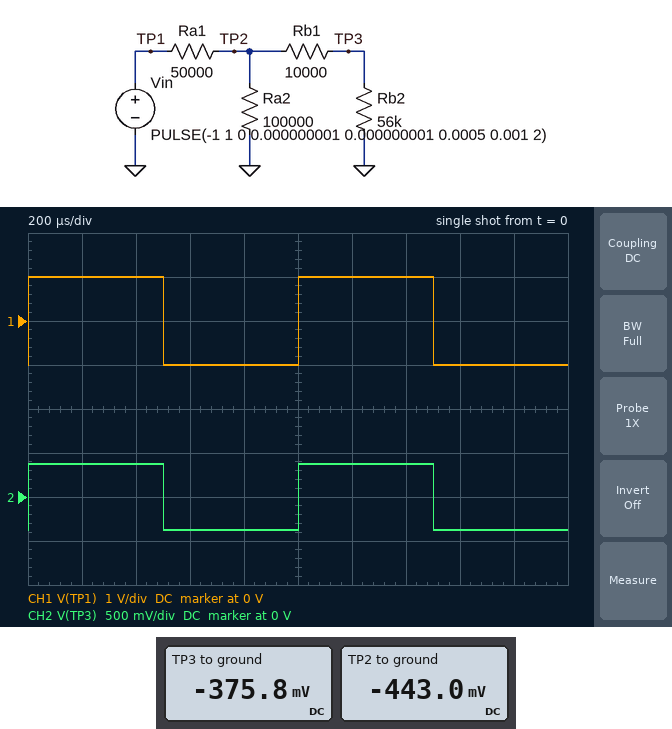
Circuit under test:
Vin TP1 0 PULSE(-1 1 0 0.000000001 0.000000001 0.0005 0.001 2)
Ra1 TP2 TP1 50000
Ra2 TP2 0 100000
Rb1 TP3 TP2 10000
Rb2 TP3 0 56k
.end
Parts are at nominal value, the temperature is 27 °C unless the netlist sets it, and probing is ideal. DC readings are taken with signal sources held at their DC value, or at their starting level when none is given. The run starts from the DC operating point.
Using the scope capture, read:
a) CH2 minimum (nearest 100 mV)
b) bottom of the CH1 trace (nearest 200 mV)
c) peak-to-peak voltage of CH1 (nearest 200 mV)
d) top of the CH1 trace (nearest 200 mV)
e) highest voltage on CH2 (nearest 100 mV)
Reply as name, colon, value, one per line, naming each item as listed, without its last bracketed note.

CH2 minimum: -400 mV
bottom of the CH1 trace: -1.0 V
peak-to-peak voltage of CH1: 2.0 V
top of the CH1 trace: 1.0 V
highest voltage on CH2: 400 mV
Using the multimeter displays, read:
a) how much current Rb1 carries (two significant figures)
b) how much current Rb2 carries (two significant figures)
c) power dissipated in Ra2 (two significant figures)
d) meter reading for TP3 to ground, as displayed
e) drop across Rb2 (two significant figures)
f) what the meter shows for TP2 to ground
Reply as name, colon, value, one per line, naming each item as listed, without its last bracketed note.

how much current Rb1 carries: 6.7 µA
how much current Rb2 carries: 6.7 µA
power dissipated in Ra2: 2.0 µW
meter reading for TP3 to ground, as displayed: -375.8 mV
drop across Rb2: 380 mV
what the meter shows for TP2 to ground: -443.0 mV
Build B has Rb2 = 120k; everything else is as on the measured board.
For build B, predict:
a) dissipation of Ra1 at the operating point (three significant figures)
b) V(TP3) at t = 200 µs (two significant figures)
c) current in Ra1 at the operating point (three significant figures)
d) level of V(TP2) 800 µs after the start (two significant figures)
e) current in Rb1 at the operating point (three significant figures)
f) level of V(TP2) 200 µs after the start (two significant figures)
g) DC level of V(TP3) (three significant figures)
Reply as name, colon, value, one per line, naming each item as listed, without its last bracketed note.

dissipation of Ra1 at the operating point: 4.41 µW
V(TP3) at t = 200 µs: 490 mV
current in Ra1 at the operating point: 9.39 µA
level of V(TP2) 800 µs after the start: -530 mV
current in Rb1 at the operating point: 4.08 µA
level of V(TP2) 200 µs after the start: 530 mV
DC level of V(TP3): -490 mV
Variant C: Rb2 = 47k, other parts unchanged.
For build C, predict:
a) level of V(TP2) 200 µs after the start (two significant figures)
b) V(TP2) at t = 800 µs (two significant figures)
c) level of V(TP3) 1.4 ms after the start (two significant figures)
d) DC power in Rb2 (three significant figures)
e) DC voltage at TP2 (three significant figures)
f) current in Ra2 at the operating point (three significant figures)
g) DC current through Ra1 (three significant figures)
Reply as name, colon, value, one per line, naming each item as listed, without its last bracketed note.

level of V(TP2) 200 µs after the start: 420 mV
V(TP2) at t = 800 µs: -420 mV
level of V(TP3) 1.4 ms after the start: 350 mV
DC power in Rb2: 2.56 µW
DC voltage at TP2: -421 mV
current in Ra2 at the operating point: 4.21 µA
DC current through Ra1: 11.6 µA
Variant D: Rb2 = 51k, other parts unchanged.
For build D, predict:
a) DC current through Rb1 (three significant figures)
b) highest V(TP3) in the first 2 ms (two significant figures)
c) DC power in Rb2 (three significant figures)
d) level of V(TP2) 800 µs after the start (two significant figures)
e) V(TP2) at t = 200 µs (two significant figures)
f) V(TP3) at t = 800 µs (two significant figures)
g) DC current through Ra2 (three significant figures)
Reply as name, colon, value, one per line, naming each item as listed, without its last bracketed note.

DC current through Rb1: 7.07 µA
highest V(TP3) in the first 2 ms: 360 mV
DC power in Rb2: 2.55 µW
level of V(TP2) 800 µs after the start: -430 mV
V(TP2) at t = 200 µs: 430 mV
V(TP3) at t = 800 µs: -360 mV
DC current through Ra2: 4.31 µA
